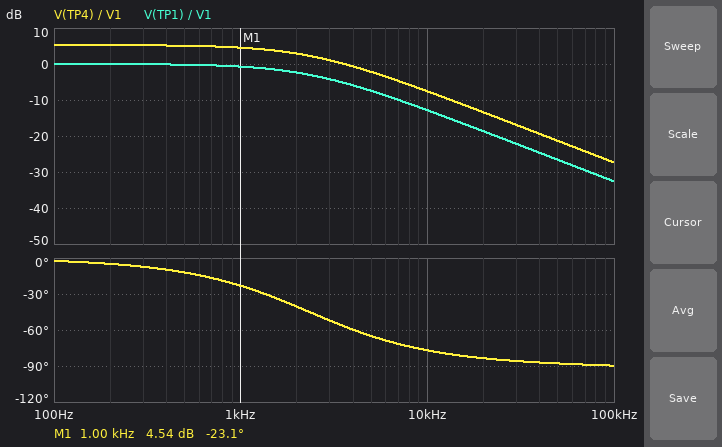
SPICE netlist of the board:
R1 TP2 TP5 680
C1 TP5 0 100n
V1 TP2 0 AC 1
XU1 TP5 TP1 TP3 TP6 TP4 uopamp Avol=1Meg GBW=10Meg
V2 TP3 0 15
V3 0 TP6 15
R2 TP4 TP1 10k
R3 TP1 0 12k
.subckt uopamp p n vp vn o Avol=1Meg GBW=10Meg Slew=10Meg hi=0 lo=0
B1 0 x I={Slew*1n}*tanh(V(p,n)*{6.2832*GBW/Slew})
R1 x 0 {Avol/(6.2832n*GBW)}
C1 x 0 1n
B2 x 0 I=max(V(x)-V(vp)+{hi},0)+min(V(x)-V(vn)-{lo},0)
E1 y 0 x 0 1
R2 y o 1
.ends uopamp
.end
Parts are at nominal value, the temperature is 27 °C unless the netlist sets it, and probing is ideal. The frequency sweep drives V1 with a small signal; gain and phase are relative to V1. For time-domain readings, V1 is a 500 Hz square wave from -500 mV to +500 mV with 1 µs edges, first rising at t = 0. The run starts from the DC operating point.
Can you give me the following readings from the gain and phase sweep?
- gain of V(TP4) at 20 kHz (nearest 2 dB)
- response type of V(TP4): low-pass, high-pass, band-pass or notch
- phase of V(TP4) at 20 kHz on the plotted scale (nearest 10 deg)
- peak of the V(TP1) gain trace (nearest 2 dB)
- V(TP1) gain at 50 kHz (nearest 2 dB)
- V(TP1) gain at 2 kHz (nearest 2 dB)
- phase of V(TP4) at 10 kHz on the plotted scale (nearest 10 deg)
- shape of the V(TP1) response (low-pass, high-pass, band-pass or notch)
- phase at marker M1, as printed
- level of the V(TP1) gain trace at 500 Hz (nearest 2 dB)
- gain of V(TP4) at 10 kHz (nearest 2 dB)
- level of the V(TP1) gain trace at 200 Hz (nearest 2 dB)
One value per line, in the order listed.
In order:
-14 dB
low-pass
-80 deg
0 dB
-26 dB
-2 dB
-80 deg
low-pass
-23.1 deg
0 dB
-8 dB
0 dB
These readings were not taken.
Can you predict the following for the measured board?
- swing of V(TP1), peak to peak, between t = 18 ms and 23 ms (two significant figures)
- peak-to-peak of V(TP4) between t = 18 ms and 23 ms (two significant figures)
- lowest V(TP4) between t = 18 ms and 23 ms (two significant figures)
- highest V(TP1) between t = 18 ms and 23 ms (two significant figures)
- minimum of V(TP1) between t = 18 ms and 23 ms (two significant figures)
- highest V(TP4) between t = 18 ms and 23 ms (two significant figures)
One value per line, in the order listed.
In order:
1.0 V
1.8 V
-920 mV
500 mV
-500 mV
920 mV
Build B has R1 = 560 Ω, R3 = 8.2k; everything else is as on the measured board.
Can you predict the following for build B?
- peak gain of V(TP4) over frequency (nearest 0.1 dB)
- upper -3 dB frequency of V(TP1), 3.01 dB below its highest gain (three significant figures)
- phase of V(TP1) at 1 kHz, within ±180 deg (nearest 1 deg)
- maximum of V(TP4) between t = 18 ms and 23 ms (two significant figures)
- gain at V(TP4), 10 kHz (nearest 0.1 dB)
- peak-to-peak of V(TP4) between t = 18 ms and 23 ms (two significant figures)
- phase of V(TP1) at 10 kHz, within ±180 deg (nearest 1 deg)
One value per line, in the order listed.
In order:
6.9 dB
2.84 kHz
-19 deg
1.1 V
-4.3 dB
2.2 V
-74 deg
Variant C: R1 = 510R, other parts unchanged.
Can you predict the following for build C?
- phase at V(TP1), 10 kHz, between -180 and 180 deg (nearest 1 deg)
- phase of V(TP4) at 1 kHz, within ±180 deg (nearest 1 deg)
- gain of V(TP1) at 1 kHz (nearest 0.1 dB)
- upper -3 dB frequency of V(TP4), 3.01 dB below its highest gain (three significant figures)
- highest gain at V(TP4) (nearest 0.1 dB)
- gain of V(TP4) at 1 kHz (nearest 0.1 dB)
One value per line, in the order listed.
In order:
-73 deg
-18 deg
-0.4 dB
3.12 kHz
5.3 dB
4.8 dB
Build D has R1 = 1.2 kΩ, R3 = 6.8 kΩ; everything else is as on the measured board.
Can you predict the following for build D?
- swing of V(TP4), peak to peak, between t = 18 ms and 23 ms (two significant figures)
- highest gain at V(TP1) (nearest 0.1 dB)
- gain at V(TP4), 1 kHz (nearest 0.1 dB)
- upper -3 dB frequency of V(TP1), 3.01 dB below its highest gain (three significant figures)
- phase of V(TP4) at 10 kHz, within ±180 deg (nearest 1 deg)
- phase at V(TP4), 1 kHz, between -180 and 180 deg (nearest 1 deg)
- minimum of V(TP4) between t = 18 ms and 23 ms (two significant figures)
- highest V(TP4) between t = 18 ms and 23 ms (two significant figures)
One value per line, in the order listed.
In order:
2.5 V
0 dB
5.9 dB
1.33 kHz
-83 deg
-37 deg
-1.2 V
1.2 V
